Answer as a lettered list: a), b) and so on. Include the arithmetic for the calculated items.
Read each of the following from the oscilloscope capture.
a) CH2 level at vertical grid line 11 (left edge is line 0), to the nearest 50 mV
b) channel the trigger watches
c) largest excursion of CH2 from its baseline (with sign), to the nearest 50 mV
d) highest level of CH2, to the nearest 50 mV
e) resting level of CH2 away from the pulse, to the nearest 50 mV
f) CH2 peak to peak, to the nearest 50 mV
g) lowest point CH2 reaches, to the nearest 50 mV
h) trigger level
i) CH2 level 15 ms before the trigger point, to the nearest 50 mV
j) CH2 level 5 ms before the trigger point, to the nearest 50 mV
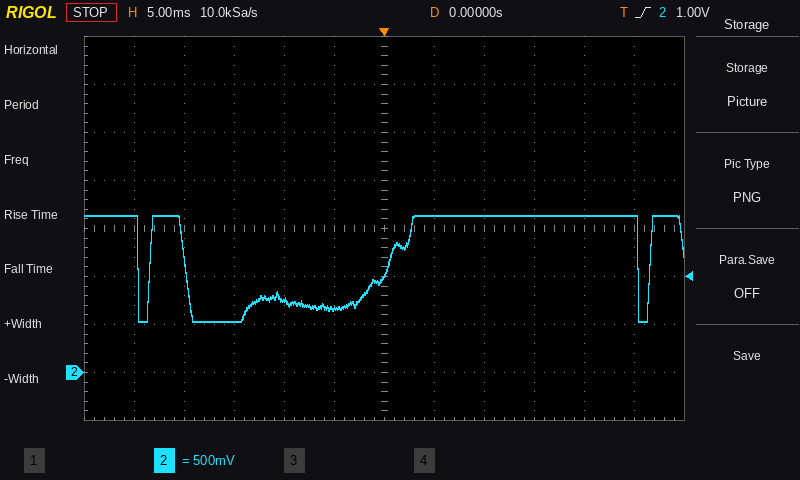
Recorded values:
a) 1.65 V
b) CH2
c) 550 mV − (1.65 V) = -1.10 V
d) 1.65 V
e) 1.65 V
f) 1.65 V − (550 mV) = 1.10 V
g) 550 mV
h) 1.00 V
i) 550 mV
j) 650 mV
